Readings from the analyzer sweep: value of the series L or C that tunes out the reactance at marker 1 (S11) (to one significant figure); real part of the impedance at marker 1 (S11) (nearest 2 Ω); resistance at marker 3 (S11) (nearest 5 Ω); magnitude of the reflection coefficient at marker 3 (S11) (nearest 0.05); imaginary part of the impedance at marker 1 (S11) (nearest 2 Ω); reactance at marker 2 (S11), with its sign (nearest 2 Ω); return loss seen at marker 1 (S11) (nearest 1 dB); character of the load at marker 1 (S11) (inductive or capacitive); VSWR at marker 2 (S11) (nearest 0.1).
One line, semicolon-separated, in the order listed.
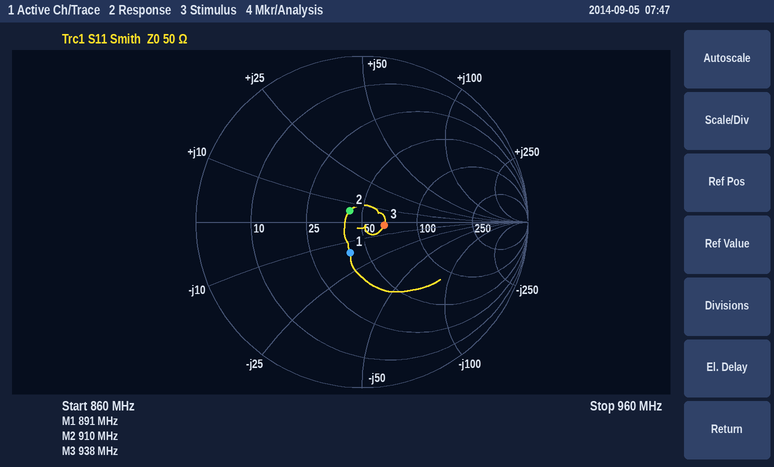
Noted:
3 nH; 40 Ω; 65 Ω; 0.15; -16 Ω; +6 Ω; 14 dB; capacitive; 1.2
